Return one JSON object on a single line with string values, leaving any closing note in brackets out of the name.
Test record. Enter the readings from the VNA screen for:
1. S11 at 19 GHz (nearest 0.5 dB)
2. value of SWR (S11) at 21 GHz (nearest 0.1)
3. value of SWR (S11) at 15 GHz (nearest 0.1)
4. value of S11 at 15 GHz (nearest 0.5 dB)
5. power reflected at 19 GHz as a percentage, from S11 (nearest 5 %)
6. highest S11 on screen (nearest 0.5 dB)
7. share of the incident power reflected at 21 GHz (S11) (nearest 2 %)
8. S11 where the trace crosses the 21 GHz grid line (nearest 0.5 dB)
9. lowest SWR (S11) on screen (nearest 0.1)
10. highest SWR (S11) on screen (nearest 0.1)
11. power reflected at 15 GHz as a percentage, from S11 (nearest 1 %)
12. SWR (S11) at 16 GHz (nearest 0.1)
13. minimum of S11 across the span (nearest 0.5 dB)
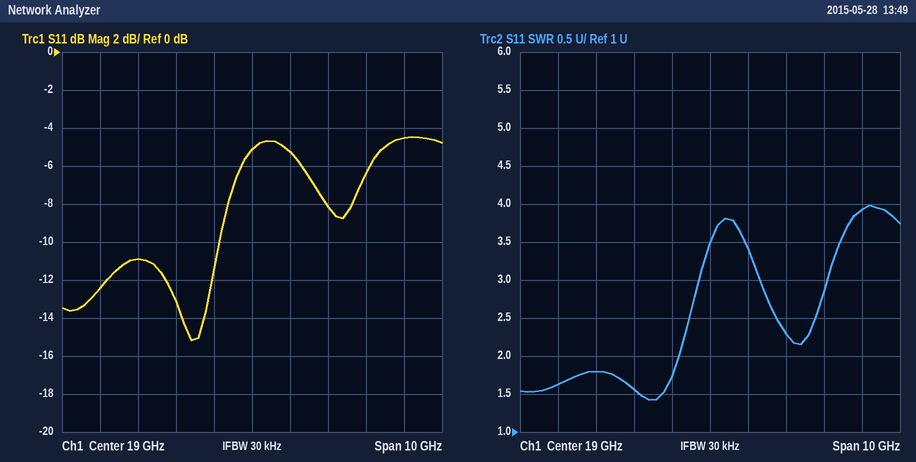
{"S11 at 19 GHz": "-5.0 dB", "value of SWR (S11) at 21 GHz": "2.3", "value of SWR (S11) at 15 GHz": "1.6", "value of S11 at 15 GHz": "-12.5 dB", "power reflected at 19 GHz as a percentage, from S11": "30 %", "highest S11 on screen": "-4.5 dB", "share of the incident power reflected at 21 GHz (S11)": "16 %", "S11 where the trace crosses the 21 GHz grid line": "-8.0 dB", "lowest SWR (S11) on screen": "1.4", "highest SWR (S11) on screen": "4.0", "power reflected at 15 GHz as a percentage, from S11": "6 %", "SWR (S11) at 16 GHz": "1.8", "minimum of S11 across the span": "-15.0 dB"}
